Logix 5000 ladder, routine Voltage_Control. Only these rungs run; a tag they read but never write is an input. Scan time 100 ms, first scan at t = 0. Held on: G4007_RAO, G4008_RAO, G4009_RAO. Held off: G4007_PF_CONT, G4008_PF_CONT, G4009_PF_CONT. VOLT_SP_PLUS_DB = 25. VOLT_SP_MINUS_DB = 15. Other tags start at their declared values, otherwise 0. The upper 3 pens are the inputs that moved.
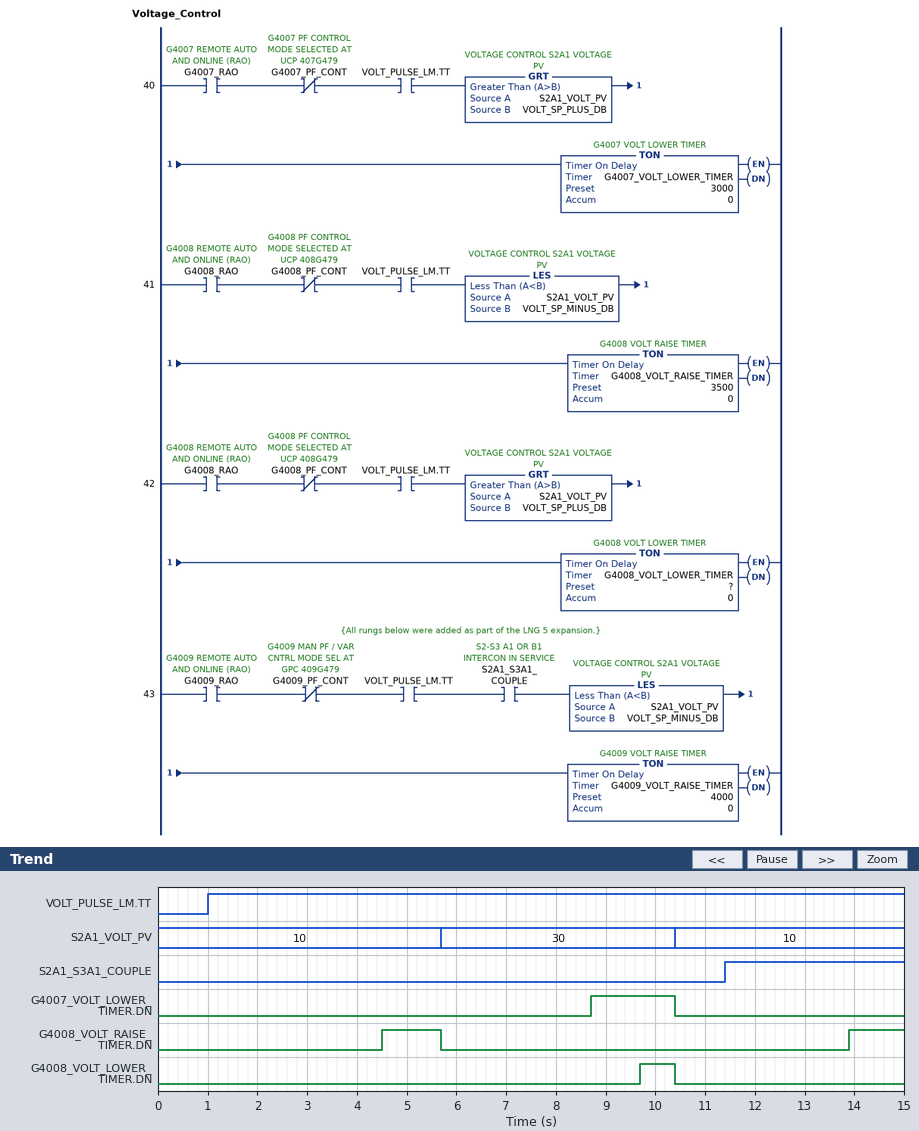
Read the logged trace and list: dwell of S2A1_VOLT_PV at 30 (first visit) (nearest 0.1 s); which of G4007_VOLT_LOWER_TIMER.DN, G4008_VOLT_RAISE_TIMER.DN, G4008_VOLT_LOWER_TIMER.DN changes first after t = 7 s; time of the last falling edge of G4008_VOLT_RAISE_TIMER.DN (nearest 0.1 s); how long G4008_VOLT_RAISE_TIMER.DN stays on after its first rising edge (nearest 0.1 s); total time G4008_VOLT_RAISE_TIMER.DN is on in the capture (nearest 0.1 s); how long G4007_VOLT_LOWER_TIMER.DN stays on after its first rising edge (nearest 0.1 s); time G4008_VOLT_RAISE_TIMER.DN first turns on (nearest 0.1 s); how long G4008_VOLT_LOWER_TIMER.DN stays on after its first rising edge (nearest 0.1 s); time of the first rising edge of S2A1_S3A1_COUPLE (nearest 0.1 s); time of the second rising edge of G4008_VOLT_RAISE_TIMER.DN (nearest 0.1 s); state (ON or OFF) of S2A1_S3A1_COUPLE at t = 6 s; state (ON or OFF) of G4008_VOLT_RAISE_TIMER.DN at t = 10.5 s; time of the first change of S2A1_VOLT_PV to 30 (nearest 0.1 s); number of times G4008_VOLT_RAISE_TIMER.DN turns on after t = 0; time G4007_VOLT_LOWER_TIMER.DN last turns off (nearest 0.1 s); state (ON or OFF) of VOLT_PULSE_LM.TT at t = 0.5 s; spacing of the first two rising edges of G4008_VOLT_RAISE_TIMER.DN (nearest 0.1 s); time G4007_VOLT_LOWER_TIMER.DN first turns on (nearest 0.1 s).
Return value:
4.7 s
G4007_VOLT_LOWER_TIMER.DN
5.7 s
1.2 s
2.3 s
1.7 s
4.5 s
0.7 s
11.4 s
13.9 s
OFF
OFF
5.7 s
2
10.4 s
OFF
9.4 s
8.7 s
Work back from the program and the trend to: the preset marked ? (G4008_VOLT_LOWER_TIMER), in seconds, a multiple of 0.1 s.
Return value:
4.0 s
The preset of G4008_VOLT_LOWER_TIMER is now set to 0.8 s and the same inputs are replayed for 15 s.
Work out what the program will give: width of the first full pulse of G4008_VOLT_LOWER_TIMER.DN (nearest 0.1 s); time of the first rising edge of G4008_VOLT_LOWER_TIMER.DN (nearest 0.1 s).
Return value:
3.9 s
6.5 s
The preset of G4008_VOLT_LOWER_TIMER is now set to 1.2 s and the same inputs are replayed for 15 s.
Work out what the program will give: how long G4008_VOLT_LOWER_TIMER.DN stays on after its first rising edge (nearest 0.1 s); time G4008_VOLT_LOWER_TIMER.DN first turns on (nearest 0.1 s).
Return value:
3.5 s
6.9 s
